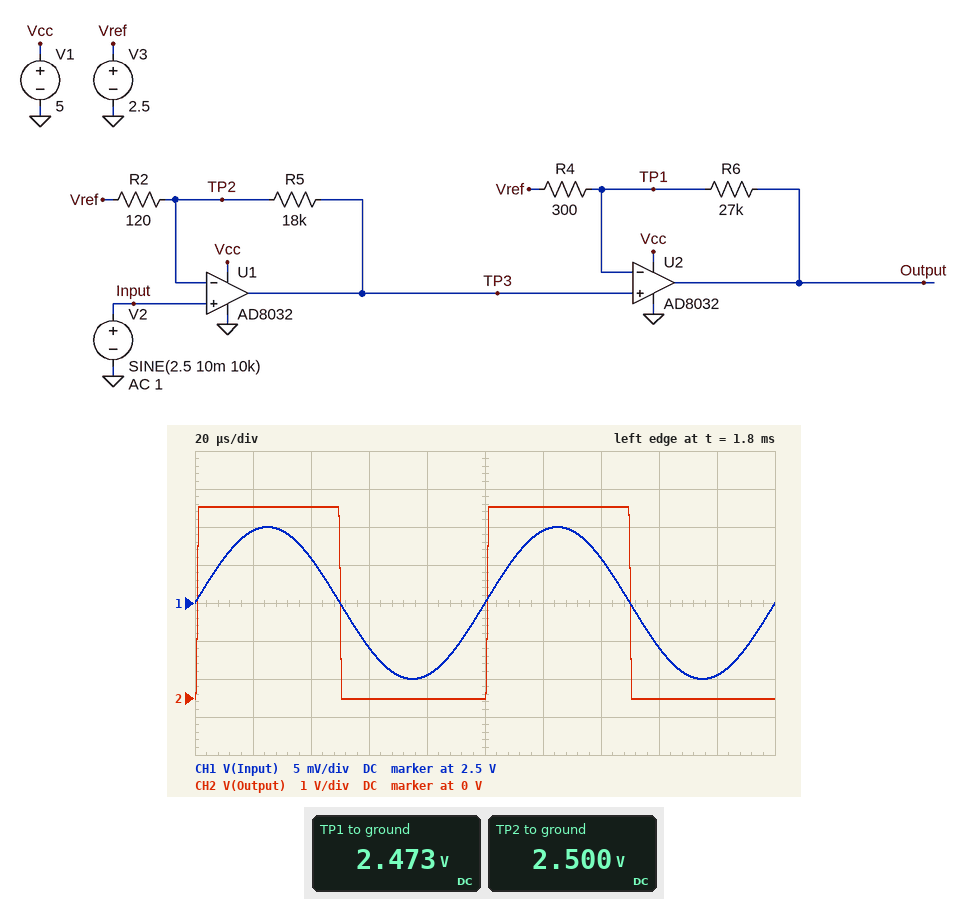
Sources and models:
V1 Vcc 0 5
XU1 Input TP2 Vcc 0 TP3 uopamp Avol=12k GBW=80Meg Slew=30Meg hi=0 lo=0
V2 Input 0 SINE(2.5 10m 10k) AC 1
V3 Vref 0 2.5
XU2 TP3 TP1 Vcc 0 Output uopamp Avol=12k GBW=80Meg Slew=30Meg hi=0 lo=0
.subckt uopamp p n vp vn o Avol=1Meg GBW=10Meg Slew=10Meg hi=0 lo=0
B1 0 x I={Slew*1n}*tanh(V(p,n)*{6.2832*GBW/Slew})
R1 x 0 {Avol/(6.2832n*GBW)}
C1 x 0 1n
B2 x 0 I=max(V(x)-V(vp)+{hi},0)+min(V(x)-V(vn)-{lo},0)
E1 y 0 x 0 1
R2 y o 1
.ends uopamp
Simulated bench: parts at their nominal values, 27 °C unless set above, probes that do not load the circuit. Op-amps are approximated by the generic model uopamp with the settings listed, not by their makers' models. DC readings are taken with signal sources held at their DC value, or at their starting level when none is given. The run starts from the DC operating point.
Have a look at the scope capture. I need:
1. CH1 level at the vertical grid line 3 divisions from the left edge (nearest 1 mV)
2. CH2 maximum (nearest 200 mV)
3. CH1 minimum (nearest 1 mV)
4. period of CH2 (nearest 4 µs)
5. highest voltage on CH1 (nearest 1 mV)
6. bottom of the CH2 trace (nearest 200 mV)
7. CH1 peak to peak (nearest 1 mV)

2.494 V
5.0 V
2.490 V
100 µs
2.510 V
0 V
20 mV
